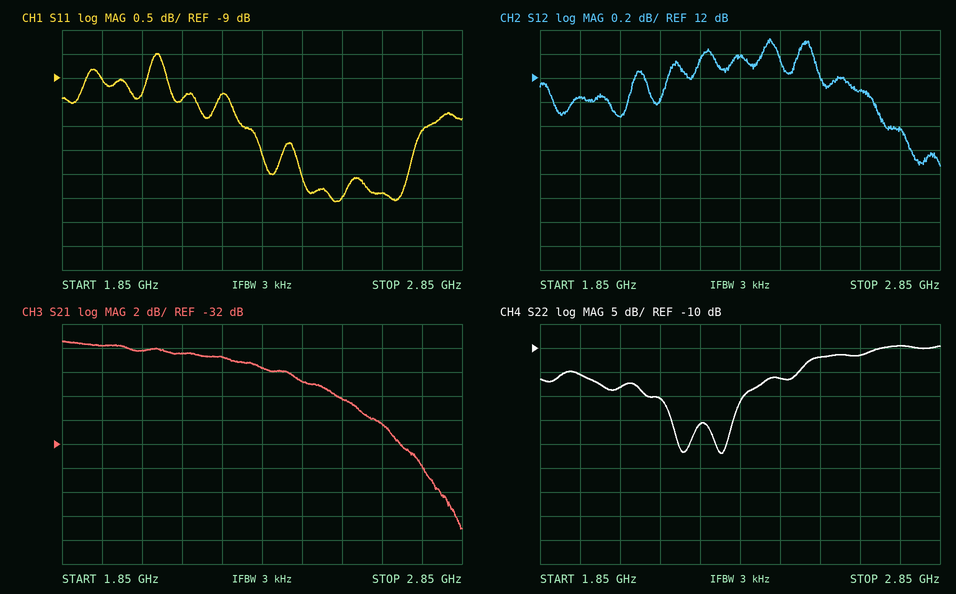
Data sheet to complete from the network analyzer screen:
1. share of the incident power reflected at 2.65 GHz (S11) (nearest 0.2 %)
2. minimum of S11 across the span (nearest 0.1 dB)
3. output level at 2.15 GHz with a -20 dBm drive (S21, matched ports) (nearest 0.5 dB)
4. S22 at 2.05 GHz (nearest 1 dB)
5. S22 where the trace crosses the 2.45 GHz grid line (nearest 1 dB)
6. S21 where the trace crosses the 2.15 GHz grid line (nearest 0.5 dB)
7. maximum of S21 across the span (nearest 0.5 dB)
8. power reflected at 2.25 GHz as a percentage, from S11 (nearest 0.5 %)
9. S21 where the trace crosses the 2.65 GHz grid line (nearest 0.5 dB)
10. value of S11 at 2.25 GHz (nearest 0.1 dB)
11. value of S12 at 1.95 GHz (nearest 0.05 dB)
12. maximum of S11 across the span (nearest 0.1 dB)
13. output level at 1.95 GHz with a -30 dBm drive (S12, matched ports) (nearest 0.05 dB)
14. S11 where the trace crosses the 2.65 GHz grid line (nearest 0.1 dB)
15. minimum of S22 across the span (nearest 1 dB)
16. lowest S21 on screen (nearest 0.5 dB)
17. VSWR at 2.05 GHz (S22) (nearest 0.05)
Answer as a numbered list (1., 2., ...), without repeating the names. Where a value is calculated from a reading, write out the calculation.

1. 10^(-11.4/10) ≈ 7.2 %
2. -11.6 dB
3. -20 dBm + (-24.5 dB) = -44.5 dBm
4. -18 dB
5. -16 dB
6. -24.5 dB
7. -23.5 dB
8. 10^(-9.3/10) ≈ 11.7 %, so 11.5 % to the nearest 0.5 %
9. -30.5 dB
10. -9.3 dB
11. 11.85 dB
12. -8.5 dB
13. -30 dBm + (11.85 dB) = -18.15 dBm
14. -11.4 dB
15. -32 dB
16. -39.0 dB
17. |Γ| = 10^(-18/20) = 0.1259; VSWR = (1 + 0.1259)/(1 − 0.1259) ≈ 1.29, so 1.30 to the nearest 0.05
